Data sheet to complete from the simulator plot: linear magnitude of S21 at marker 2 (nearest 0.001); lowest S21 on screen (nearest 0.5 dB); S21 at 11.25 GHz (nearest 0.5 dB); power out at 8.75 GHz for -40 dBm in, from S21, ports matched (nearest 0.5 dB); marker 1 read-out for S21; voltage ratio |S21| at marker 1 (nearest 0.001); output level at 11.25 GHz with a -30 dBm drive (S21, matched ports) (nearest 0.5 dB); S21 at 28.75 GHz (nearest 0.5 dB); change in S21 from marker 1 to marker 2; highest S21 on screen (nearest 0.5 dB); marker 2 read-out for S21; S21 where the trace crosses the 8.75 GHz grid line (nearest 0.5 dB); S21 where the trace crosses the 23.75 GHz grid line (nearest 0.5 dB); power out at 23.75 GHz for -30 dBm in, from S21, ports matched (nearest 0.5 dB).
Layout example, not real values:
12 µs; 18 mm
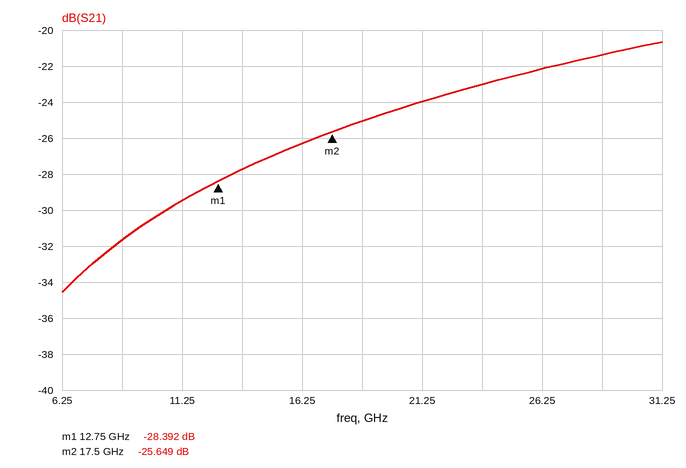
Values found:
0.052; -34.5 dB; -29.5 dB; -71.5 dBm; -28.392 dB; 0.038; -59.5 dBm; -21.5 dB; 2.743 dB; -20.5 dB; -25.649 dB; -31.5 dB; -23.0 dB; -53.0 dBm
